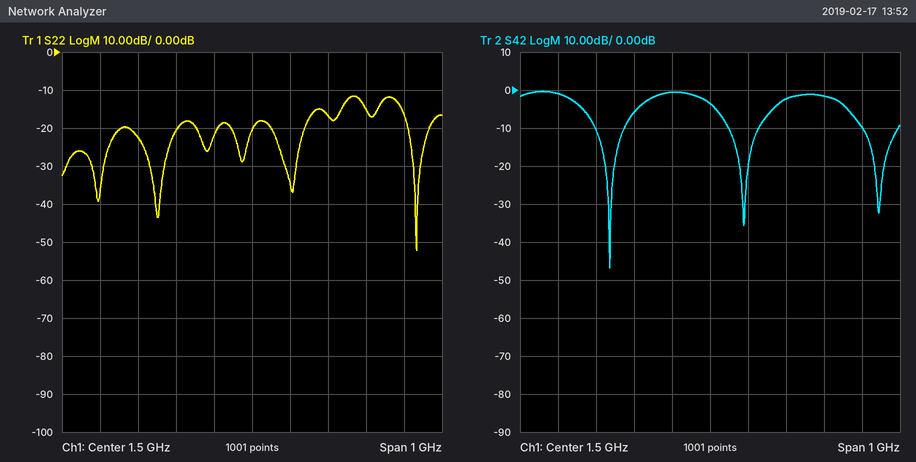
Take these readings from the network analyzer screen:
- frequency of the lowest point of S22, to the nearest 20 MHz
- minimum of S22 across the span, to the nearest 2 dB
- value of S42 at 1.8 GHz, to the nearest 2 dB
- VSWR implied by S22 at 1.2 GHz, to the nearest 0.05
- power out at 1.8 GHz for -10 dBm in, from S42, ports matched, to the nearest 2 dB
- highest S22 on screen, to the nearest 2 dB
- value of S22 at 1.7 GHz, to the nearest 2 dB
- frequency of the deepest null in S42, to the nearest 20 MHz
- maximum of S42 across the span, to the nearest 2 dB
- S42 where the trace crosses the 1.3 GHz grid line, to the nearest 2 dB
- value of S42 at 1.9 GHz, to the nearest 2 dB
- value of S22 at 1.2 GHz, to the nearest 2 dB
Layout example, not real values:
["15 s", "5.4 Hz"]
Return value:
["1.94 GHz", "-52 dB", "-2 dB", "1.15", "-12 dBm", "-12 dB", "-16 dB", "1.24 GHz", "0 dB", "-6 dB", "-10 dB", "-22 dB"]
